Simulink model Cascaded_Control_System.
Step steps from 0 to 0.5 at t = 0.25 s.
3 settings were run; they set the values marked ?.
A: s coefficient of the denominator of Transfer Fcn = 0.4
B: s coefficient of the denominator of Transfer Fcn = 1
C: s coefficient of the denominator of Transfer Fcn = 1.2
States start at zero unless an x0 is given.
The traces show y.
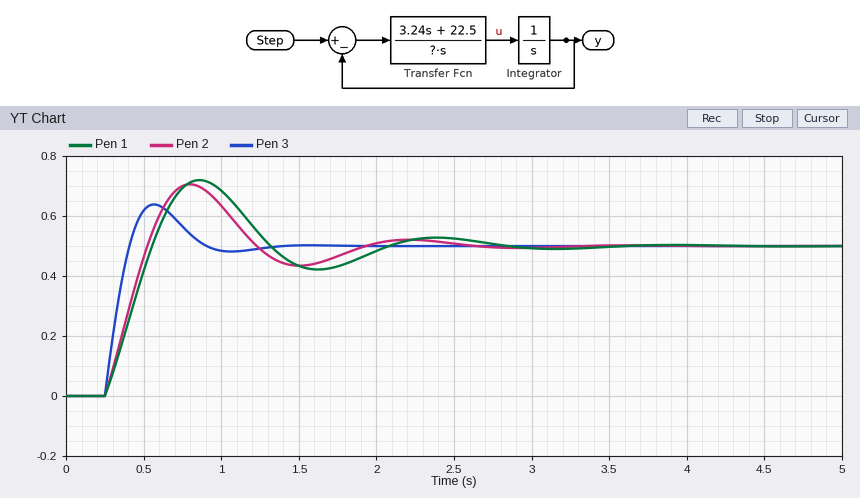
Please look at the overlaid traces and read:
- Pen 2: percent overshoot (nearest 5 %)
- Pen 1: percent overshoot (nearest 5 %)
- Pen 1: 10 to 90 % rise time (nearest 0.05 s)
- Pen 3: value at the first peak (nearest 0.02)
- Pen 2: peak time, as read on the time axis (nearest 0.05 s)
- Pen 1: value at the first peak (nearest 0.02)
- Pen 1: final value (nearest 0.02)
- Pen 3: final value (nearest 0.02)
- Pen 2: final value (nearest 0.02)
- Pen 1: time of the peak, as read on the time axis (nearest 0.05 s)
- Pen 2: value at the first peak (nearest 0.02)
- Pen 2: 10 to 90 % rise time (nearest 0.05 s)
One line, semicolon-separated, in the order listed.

40 %; 45 %; 0.25 s; 0.64; 0.80 s; 0.72; 0.50; 0.50; 0.50; 0.85 s; 0.70; 0.20 s
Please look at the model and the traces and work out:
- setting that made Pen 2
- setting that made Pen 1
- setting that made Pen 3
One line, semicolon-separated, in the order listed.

B; C; A
